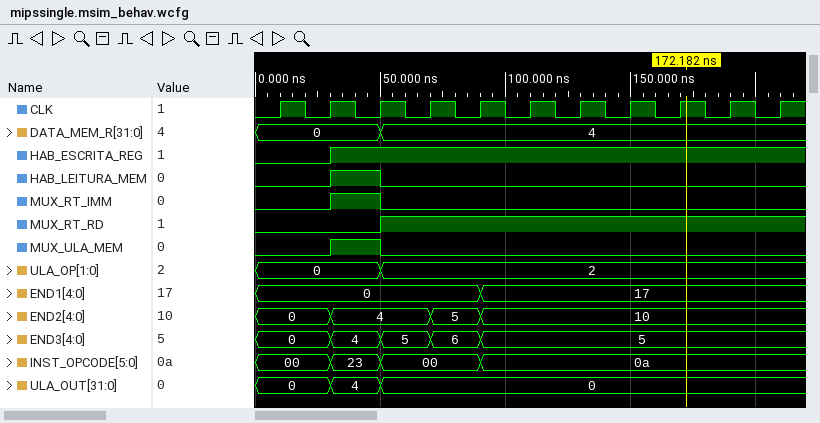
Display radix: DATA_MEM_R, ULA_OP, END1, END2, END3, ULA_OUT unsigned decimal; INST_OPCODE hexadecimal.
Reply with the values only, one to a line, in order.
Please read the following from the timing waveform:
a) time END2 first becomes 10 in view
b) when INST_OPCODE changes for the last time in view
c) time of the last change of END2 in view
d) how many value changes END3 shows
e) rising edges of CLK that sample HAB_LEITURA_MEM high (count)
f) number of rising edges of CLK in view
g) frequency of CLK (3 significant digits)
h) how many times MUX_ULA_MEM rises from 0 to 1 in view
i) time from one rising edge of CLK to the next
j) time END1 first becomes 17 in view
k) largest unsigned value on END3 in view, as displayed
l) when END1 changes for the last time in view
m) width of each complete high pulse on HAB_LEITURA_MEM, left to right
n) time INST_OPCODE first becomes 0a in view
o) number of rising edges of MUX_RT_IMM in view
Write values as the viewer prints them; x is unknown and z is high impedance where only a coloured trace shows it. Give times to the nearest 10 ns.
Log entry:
90 ns
90 ns
90 ns
4
1
11
50.0 MHz
1
20 ns
90 ns
6
90 ns
20 ns
90 ns
1
